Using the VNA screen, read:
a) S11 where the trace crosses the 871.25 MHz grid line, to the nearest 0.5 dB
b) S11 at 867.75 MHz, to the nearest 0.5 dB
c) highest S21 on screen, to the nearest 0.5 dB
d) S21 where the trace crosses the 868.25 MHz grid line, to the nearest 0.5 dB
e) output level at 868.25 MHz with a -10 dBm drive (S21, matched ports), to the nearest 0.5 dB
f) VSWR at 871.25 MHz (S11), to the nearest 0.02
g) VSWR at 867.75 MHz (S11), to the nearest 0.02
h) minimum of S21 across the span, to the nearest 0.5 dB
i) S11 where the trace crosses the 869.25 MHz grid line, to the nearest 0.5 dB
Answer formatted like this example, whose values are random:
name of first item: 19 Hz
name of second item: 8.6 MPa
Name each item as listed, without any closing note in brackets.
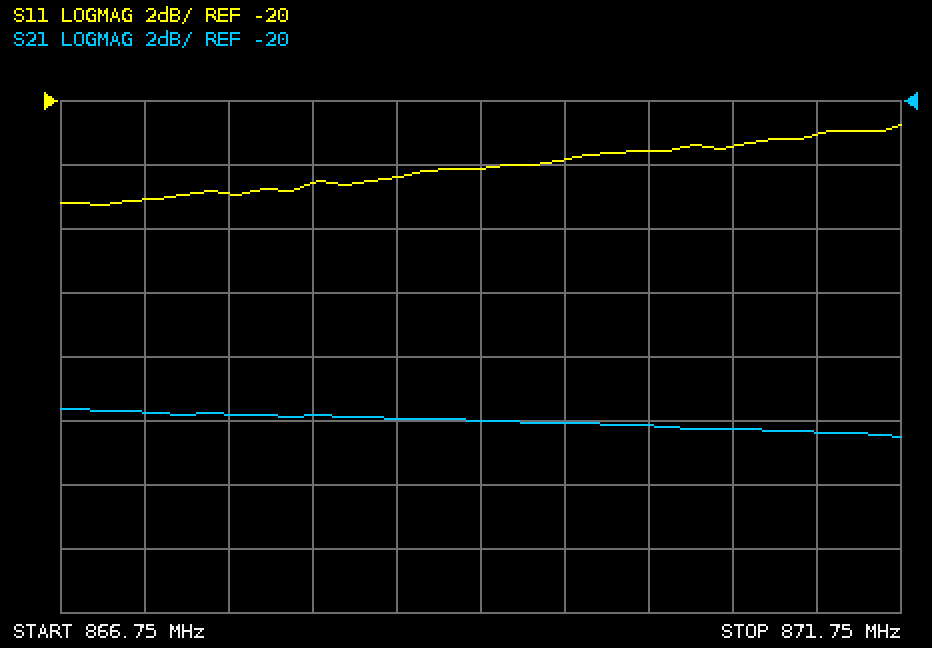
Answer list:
S11 where the trace crosses the 871.25 MHz grid line, to the nearest 0.5 dB: -21.0 dB
S11 at 867.75 MHz, to the nearest 0.5 dB: -23.0 dB
highest S21 on screen, to the nearest 0.5 dB: -29.5 dB
S21 where the trace crosses the 868.25 MHz grid line, to the nearest 0.5 dB: -30.0 dB
output level at 868.25 MHz with a -10 dBm drive (S21, matched ports), to the nearest 0.5 dB: -40.0 dBm
VSWR at 871.25 MHz (S11), to the nearest 0.02: 1.20
VSWR at 867.75 MHz (S11), to the nearest 0.02: 1.16
minimum of S21 across the span, to the nearest 0.5 dB: -30.5 dB
S11 where the trace crosses the 869.25 MHz grid line, to the nearest 0.5 dB: -22.0 dB
